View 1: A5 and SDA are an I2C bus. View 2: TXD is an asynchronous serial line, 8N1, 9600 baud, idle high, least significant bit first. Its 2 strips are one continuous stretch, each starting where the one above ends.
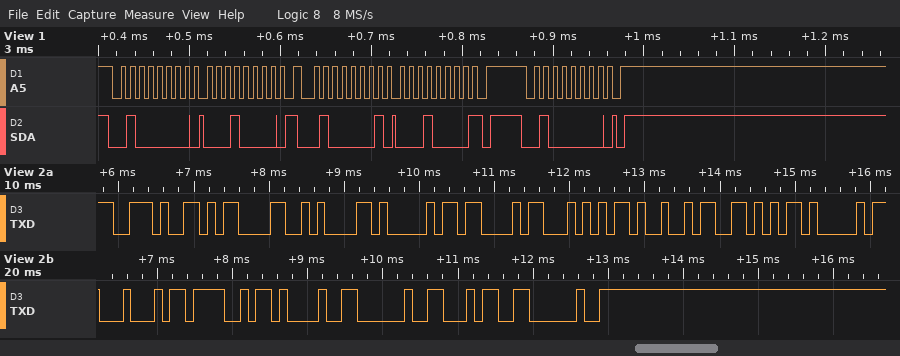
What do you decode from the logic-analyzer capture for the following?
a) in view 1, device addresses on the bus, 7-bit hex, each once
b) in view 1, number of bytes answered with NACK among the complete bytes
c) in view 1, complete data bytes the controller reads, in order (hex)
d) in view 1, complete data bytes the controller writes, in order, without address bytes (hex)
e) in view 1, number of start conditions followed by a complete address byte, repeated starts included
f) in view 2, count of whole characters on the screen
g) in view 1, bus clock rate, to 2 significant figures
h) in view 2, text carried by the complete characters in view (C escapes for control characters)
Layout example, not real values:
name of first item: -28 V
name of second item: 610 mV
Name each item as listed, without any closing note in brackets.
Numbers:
in view 1, device addresses on the bus, 7-bit hex, each once: 0x20
in view 1, number of bytes answered with NACK among the complete bytes: 1
in view 1, complete data bytes the controller reads, in order: 10
in view 1, complete data bytes the controller writes, in order, without address bytes: 10
in view 1, number of start conditions followed by a complete address byte, repeated starts included: 3
in view 2, count of whole characters on the screen: 15
in view 1, bus clock rate, to 2 significant figures: 100 kHz
in view 2, text carried by the complete characters in view: ".\r\nACTIVADO! 4 "
